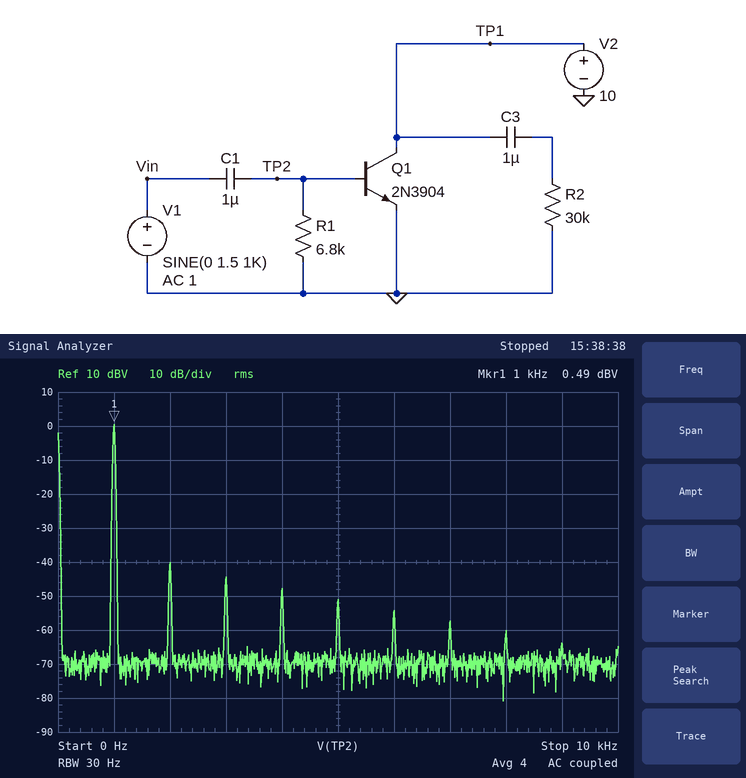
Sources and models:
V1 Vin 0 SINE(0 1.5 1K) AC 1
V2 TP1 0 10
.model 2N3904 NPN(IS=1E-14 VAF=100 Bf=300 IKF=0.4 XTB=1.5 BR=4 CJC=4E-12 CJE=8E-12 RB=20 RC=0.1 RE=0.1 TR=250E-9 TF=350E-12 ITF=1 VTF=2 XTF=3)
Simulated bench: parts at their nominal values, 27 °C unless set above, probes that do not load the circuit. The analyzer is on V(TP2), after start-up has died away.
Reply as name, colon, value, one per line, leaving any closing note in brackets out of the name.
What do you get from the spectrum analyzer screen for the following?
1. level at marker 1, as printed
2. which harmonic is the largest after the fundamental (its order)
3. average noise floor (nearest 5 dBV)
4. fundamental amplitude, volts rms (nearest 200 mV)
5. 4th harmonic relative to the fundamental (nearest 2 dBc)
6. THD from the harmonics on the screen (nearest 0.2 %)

level at marker 1, as printed: 0.49 dBV
which harmonic is the largest after the fundamental: 2
average noise floor: -70 dBV
fundamental amplitude, volts rms: 1.0 V
4th harmonic relative to the fundamental: -48 dBc
THD from the harmonics on the screen: 1.2 %
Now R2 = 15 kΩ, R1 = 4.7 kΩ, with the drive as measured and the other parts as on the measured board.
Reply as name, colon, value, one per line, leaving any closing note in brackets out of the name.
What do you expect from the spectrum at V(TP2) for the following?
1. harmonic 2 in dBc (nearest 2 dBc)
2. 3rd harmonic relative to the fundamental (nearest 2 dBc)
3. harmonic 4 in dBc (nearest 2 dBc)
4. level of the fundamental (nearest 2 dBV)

harmonic 2 in dBc: -38 dBc
3rd harmonic relative to the fundamental: -42 dBc
harmonic 4 in dBc: -46 dBc
level of the fundamental: 0 dBV
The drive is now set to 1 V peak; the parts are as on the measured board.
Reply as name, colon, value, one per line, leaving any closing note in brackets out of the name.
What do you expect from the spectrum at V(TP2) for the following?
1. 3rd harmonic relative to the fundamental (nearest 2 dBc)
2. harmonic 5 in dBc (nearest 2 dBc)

3rd harmonic relative to the fundamental: -52 dBc
harmonic 5 in dBc: -58 dBc
